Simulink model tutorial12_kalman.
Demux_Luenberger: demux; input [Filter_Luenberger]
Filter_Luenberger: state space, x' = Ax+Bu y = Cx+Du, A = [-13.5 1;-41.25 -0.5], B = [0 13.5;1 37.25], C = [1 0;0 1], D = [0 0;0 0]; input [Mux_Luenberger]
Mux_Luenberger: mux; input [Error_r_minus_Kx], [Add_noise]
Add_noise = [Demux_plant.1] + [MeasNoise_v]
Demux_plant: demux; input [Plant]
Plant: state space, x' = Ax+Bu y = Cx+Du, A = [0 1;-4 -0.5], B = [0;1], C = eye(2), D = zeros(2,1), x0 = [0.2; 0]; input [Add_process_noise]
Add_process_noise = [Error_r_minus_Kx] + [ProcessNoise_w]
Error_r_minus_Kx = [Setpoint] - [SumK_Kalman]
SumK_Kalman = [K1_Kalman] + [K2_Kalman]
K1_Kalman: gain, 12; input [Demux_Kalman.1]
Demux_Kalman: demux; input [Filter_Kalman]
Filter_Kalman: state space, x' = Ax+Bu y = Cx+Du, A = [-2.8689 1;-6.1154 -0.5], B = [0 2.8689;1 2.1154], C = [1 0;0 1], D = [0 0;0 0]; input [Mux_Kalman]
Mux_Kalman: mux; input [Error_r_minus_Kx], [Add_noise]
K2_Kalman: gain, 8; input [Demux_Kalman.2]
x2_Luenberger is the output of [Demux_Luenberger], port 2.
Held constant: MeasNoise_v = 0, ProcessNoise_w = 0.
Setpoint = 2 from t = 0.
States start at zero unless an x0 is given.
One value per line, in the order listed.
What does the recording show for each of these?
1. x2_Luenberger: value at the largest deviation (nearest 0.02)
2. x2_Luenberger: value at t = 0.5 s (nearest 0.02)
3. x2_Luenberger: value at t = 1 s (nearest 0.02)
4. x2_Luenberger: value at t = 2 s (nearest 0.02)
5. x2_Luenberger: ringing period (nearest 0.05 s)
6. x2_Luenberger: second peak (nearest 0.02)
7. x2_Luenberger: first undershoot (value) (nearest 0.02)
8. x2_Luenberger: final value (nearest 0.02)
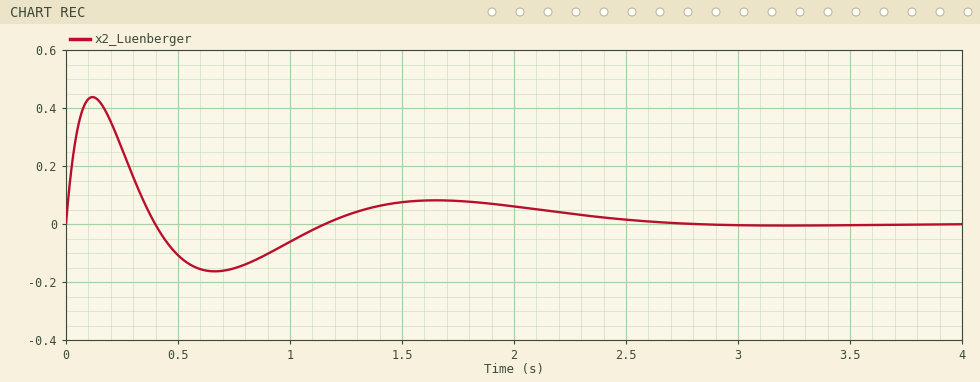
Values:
0.44
-0.10
-0.06
0.06
1.55 s
0.08
-0.16
0.00
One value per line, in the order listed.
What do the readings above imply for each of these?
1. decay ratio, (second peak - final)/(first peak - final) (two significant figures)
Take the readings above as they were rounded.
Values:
0.18
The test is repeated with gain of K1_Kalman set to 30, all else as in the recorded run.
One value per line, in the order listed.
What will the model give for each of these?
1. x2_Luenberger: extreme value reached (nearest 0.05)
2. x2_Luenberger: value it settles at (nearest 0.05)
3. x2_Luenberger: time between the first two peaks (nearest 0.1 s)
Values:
0.40
0.00
1.3 s
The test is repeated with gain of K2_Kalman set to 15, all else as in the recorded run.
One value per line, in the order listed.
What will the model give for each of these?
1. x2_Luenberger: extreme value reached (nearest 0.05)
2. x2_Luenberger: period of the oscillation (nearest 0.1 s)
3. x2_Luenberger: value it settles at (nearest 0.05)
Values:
0.40
1.6 s
0.00
